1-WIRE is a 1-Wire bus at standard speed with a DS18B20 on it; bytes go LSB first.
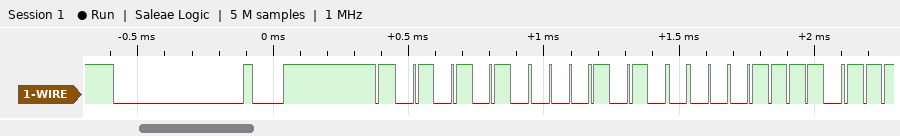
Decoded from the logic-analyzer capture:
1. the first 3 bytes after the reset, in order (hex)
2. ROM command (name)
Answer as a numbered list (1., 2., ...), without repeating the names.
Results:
1. 55 28 78
2. Match ROM
